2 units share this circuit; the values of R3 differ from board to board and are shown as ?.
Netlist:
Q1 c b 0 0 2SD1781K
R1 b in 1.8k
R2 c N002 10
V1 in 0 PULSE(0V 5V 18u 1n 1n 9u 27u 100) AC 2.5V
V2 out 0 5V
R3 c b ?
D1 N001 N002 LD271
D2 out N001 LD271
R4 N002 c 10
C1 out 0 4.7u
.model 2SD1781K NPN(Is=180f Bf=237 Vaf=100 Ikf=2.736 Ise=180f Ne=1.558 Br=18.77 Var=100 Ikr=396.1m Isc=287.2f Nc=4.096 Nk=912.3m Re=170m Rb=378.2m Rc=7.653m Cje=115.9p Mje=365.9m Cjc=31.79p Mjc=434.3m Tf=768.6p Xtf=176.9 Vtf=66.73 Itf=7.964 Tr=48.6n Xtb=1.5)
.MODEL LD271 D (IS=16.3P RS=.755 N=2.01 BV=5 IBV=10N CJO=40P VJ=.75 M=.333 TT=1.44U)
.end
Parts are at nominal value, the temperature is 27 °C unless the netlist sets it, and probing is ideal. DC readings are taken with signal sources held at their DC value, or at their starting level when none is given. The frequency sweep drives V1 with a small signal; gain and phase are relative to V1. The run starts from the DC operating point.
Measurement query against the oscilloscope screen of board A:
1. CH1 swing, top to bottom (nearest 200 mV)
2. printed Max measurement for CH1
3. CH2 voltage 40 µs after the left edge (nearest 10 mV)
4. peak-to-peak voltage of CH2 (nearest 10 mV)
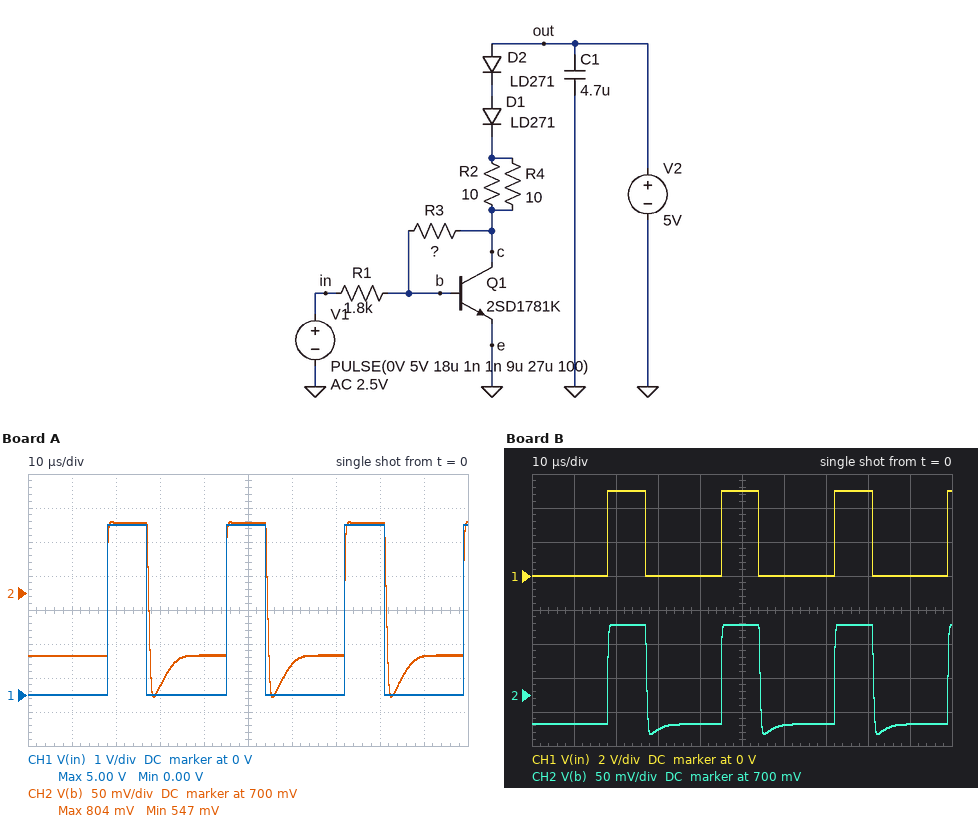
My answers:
5.0 V
5.00 V
610 mV
260 mV
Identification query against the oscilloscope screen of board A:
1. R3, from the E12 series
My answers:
6.8 kΩ
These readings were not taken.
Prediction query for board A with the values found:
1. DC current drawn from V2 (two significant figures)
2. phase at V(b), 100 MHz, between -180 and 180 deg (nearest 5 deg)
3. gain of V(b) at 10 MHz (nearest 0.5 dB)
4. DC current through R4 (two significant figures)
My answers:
3.3 mA
-85 deg
-30.5 dB
1.6 mA
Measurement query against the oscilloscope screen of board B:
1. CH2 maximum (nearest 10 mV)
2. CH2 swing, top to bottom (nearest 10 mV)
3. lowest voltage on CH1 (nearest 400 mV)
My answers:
800 mV
160 mV
0 V
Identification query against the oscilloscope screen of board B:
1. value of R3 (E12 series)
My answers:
4.7 kΩ
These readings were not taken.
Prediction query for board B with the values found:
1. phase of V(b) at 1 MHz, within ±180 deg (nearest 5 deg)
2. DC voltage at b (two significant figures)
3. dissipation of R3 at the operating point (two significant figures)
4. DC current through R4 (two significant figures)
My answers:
-45 deg
660 mV
910 µW
8.8 mA
